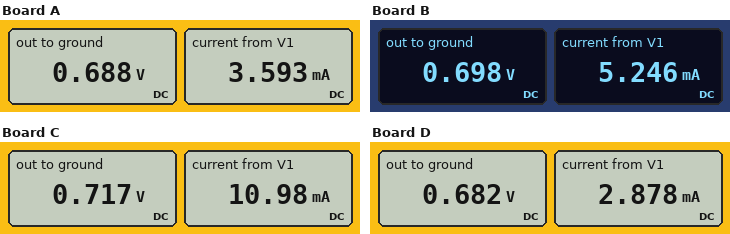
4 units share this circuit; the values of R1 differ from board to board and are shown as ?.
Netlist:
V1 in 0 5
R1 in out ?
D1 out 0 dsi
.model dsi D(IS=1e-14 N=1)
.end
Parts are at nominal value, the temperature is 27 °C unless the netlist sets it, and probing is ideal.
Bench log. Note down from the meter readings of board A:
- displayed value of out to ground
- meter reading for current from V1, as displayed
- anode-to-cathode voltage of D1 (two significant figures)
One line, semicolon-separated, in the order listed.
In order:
0.688 V; 3.593 mA; 690 mV
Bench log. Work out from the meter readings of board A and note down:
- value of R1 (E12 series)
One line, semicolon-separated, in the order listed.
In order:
1.2 kΩ
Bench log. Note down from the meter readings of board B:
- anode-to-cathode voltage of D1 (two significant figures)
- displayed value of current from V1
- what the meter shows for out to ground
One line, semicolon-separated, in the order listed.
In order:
700 mV; 5.246 mA; 0.698 V
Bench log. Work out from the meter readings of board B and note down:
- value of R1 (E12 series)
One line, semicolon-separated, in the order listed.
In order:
820 Ω
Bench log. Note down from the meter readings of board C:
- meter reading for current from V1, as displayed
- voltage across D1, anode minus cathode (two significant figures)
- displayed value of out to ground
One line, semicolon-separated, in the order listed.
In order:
10.98 mA; 720 mV; 0.717 V
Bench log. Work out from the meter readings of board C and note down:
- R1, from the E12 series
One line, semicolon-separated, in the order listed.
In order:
390 Ω
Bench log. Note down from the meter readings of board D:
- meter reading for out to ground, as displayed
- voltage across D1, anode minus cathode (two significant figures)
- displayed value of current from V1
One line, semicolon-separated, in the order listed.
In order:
0.682 V; 680 mV; 2.878 mA
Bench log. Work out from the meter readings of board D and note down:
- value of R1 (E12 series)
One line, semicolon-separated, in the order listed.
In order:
1.5 kΩ
